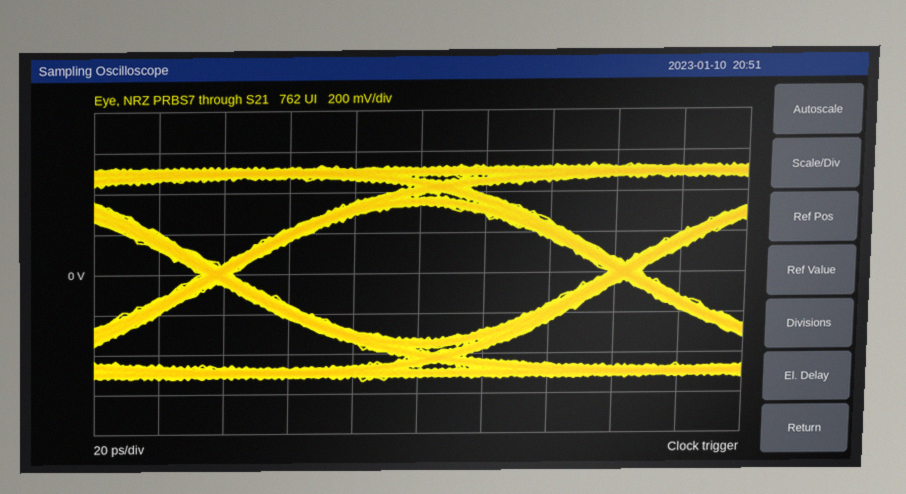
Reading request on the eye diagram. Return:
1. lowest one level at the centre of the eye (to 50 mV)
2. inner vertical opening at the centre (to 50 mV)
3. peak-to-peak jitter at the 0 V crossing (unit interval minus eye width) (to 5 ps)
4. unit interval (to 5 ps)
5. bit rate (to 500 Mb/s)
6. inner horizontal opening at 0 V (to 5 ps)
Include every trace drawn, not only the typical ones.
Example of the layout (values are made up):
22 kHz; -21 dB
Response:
350 mV; 650 mV; 10 ps; 125 ps; 8.0 Gb/s; 115 ps
